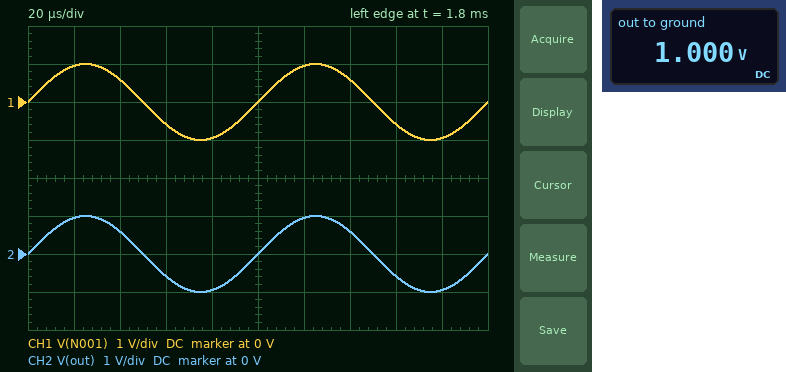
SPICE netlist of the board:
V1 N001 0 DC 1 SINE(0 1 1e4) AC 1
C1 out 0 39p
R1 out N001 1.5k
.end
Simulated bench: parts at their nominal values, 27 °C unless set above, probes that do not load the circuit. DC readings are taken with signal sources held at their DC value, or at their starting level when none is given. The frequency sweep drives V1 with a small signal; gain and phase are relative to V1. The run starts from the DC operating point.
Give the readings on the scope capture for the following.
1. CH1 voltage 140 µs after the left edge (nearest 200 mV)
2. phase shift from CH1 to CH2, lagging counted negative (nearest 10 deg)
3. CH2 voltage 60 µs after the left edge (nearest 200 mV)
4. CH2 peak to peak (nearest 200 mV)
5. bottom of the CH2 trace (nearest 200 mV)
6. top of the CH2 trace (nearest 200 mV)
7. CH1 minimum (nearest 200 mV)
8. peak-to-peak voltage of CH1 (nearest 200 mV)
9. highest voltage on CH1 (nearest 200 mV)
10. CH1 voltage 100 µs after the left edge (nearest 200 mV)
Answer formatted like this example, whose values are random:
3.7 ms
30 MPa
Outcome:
600 mV
0 deg
-600 mV
2.0 V
-1.0 V
1.0 V
-1.0 V
2.0 V
1.0 V
0 V
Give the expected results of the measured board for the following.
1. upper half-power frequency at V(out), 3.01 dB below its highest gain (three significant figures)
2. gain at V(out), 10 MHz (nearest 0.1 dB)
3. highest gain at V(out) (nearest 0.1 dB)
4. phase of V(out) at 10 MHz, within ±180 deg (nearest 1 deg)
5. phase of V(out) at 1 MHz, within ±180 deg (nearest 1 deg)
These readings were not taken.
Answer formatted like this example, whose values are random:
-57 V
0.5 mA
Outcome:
2.72 MHz
-11.6 dB
0 dB
-75 deg
-20 deg
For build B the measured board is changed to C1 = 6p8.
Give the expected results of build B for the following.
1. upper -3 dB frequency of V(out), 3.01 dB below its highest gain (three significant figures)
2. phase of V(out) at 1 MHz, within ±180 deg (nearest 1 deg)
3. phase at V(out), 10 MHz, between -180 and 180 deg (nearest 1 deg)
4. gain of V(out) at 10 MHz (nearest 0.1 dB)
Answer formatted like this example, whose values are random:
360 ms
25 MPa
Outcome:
15.6 MHz
-4 deg
-33 deg
-1.5 dB
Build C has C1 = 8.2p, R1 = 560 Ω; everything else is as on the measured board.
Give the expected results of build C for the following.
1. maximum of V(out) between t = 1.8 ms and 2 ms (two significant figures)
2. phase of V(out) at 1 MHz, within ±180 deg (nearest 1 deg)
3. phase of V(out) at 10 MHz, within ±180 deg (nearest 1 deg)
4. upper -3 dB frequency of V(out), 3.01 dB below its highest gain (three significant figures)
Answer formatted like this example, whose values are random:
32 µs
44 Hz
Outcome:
1.0 V
-2 deg
-16 deg
34.7 MHz
